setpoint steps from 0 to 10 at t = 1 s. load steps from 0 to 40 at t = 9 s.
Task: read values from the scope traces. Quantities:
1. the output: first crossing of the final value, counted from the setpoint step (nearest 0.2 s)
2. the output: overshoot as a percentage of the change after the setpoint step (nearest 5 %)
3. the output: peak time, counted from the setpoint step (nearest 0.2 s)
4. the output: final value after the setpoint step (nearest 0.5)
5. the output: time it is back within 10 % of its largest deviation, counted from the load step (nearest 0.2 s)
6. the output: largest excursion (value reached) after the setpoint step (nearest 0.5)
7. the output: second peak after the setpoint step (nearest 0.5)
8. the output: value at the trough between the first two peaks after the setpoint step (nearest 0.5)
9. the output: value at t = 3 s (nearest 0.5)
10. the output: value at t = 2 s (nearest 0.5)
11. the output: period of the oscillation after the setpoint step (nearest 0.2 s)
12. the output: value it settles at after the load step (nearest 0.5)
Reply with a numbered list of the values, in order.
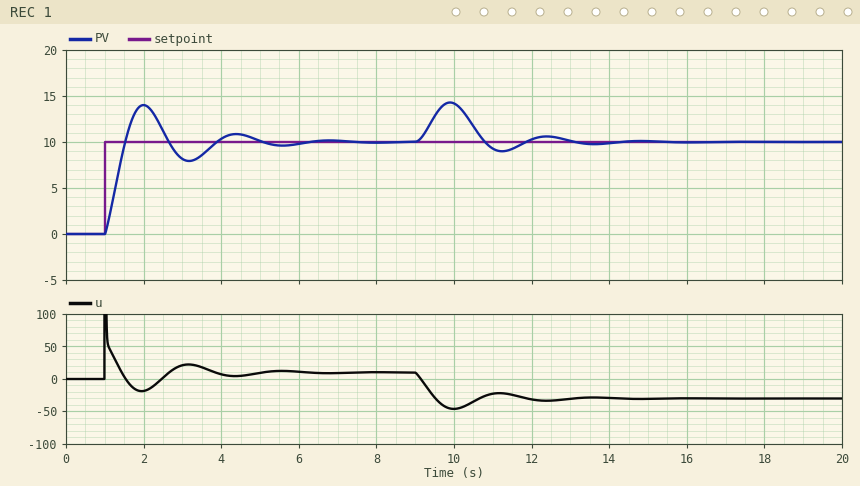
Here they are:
1. 0.6 s
2. 40 %
3. 1.0 s
4. 10.0
5. 3.8 s
6. 14.0
7. 11.0
8. 8.0
9. 8.0
10. 14.0
11. 2.4 s
12. 10.0
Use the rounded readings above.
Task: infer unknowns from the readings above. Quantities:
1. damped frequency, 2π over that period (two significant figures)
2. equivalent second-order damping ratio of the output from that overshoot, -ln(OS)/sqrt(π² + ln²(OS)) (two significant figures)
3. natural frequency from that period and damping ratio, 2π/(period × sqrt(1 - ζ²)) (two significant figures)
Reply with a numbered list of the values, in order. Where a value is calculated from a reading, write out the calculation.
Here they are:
1. 2π / 2.4 = 2.6 rad/s
2. ln(0.4) = -0.916; 0.916 / sqrt(9.870 + 0.840) = 0.28
3. 2π / (2.4 × sqrt(1 - 0.28²)) = 2.7 rad/s
